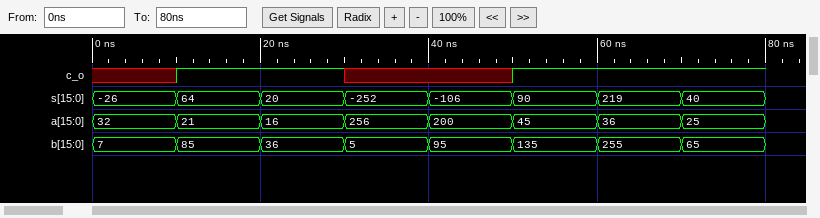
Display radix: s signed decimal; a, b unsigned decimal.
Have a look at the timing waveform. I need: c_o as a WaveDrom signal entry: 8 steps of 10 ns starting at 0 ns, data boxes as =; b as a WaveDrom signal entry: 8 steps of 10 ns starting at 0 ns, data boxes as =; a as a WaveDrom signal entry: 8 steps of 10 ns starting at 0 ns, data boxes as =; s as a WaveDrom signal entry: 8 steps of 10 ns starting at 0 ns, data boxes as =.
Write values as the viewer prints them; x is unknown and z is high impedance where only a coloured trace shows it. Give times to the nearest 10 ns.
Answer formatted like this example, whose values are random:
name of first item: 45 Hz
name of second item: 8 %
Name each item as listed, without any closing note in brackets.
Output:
c_o as a WaveDrom signal entry: 8 steps of 10 ns starting at 0 ns, data boxes as =: {name: 'c_o', wave: 'x1.x.1..'}
b as a WaveDrom signal entry: 8 steps of 10 ns starting at 0 ns, data boxes as =: {name: 'b', wave: '========', data: '7 85 36 5 95 135 255 65'}
a as a WaveDrom signal entry: 8 steps of 10 ns starting at 0 ns, data boxes as =: {name: 'a', wave: '========', data: '32 21 16 256 200 45 36 25'}
s as a WaveDrom signal entry: 8 steps of 10 ns starting at 0 ns, data boxes as =: {name: 's', wave: '========', data: '-26 64 20 -252 -106 90 219 40'}
